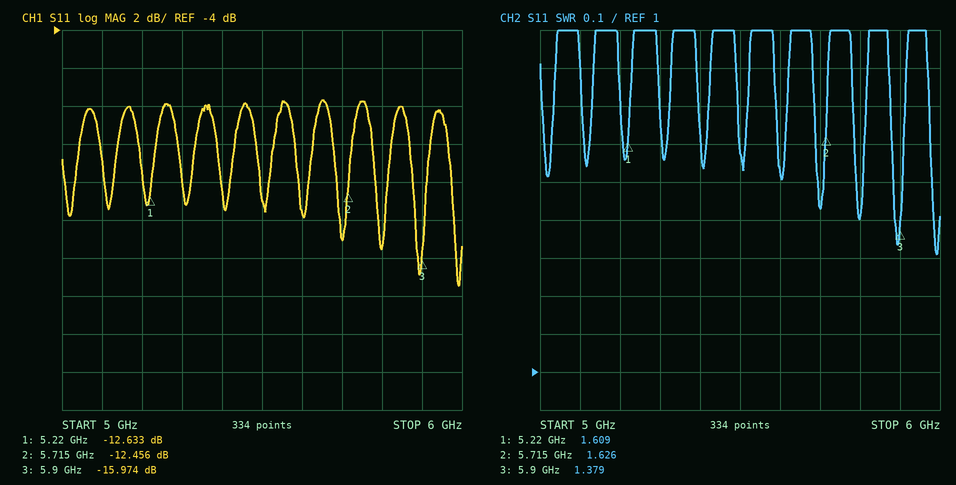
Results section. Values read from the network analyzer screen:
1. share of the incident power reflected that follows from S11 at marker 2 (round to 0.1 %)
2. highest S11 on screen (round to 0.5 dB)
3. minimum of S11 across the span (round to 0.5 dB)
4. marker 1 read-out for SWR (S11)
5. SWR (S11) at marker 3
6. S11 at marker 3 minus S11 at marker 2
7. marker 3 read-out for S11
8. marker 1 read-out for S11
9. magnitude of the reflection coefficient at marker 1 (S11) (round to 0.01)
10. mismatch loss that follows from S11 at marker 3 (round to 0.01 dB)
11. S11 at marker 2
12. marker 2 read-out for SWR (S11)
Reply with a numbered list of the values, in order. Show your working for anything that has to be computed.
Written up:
1. 10^(-12.456/10) ≈ 5.7 %
2. -7.5 dB
3. -17.5 dB
4. 1.609
5. 1.379
6. -15.974 − (-12.456) = -3.518 dB
7. -15.974 dB
8. -12.633 dB
9. 10^(-12.633/20) ≈ 0.23
10. −10 log10(1 − 10^(-15.974/10)) ≈ 0.11 dB
11. -12.456 dB
12. 1.626
